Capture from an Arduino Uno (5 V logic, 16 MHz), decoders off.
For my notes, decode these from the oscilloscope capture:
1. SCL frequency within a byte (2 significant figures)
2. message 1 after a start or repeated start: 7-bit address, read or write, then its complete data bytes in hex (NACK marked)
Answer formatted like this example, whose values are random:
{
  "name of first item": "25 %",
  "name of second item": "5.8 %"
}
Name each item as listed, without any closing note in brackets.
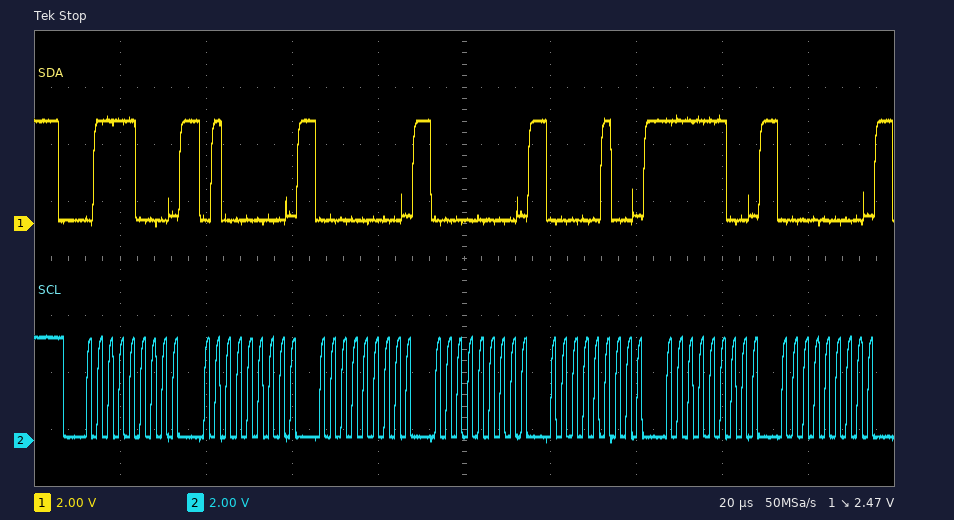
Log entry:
{
  "SCL frequency within a byte": "400 kHz",
  "message 1 after a start or repeated start: 7-bit address, read or write, then its complete data bytes in hex": "0x3C write: 40 00 00 04 FC 00"
}
